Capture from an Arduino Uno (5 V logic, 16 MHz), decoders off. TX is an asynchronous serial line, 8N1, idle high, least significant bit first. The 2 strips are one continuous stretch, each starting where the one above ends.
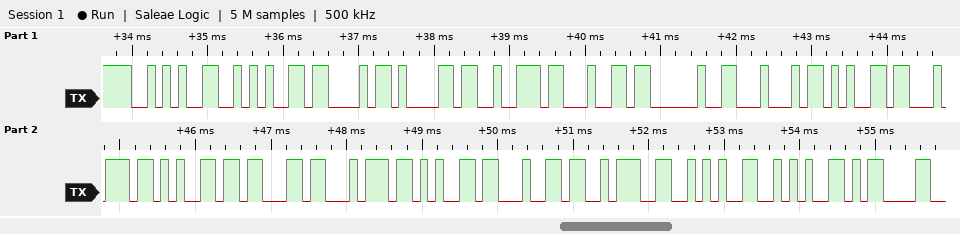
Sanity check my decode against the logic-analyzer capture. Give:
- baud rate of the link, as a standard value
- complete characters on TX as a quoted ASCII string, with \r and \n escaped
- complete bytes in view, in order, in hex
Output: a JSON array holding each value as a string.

["9600 baud", "\"**Card Detected:**\\r\"", "2A 2A 43 61 72 64 20 44 65 74 65 63 74 65 64 3A 2A 2A 0D"]
